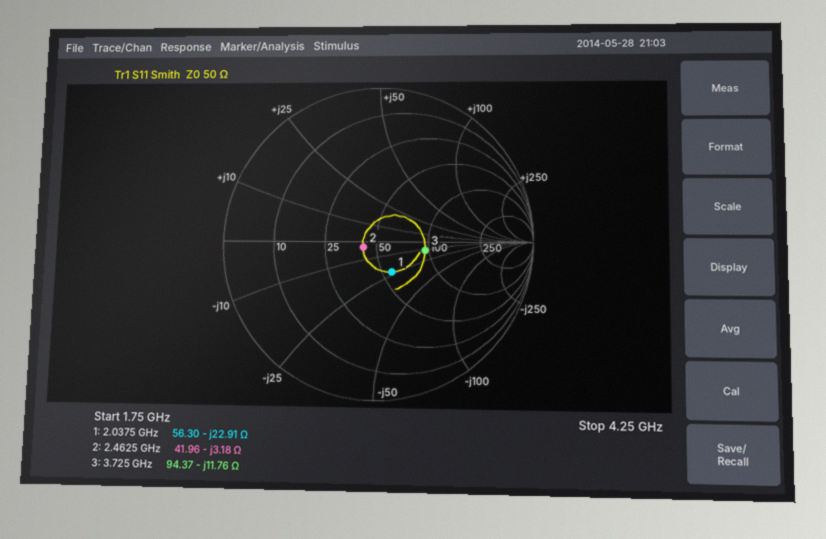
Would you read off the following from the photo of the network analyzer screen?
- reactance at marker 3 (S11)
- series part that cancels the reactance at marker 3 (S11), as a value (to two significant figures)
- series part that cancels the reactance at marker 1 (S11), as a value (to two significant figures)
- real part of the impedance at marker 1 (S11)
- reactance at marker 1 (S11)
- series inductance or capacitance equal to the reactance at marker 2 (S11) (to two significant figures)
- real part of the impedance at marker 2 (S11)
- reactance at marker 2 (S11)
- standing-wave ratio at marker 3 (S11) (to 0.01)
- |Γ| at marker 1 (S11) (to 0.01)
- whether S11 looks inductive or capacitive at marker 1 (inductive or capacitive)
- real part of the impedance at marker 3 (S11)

-11.76 Ω
500 pH
1.8 nH
56.30 Ω
-22.91 Ω
20 pF
41.96 Ω
-3.18 Ω
1.93
0.22
capacitive
94.37 Ω
